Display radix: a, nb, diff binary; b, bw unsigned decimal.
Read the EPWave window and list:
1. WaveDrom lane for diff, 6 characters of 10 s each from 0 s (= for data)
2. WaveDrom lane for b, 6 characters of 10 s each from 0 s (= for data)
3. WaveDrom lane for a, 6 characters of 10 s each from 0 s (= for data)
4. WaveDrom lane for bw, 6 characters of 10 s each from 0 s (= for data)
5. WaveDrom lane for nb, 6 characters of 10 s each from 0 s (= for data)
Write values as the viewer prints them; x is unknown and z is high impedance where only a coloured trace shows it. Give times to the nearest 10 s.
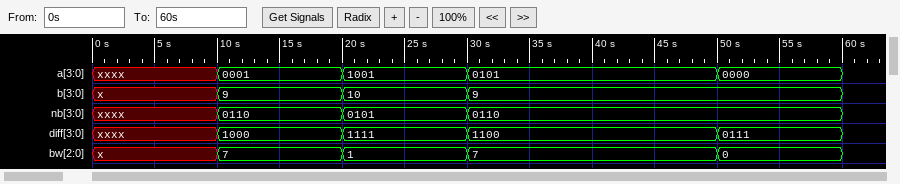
{name: 'diff', wave: 'x===.=', data: '1000 1111 1100 0111'}
{name: 'b', wave: 'x===..', data: '9 10 9'}
{name: 'a', wave: 'x===.=', data: '0001 1001 0101 0000'}
{name: 'bw', wave: 'x===.=', data: '7 1 7 0'}
{name: 'nb', wave: 'x===..', data: '0110 0101 0110'}
